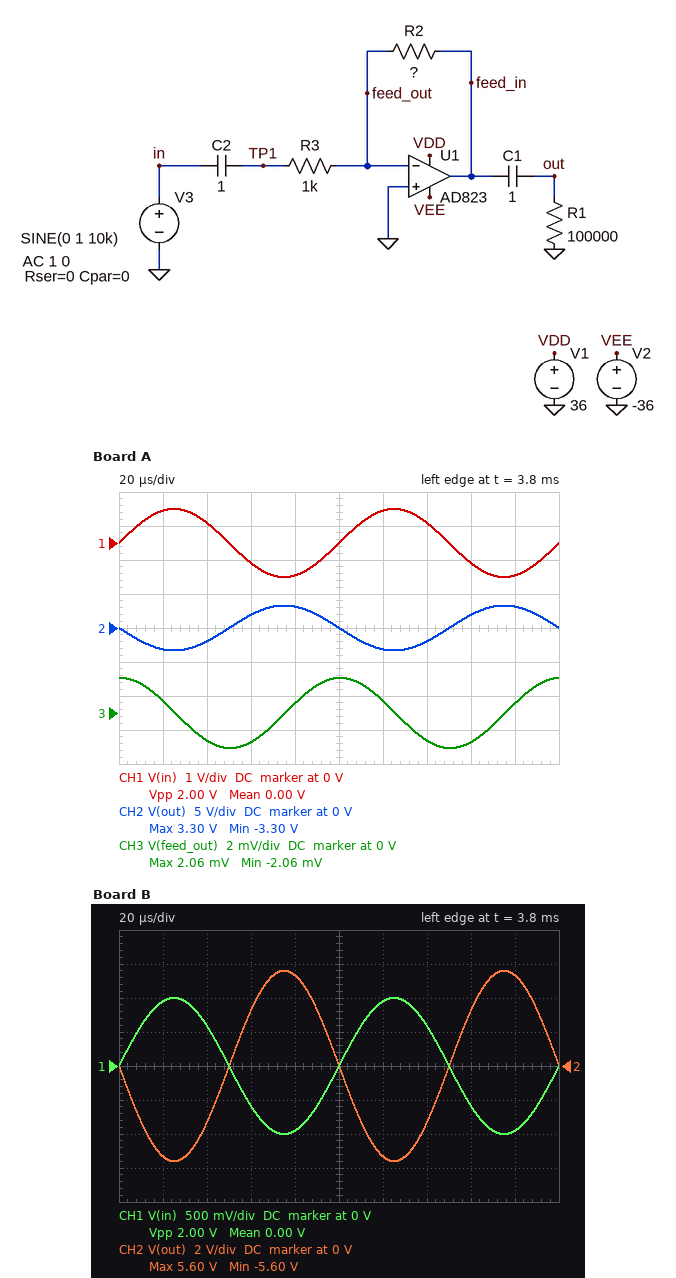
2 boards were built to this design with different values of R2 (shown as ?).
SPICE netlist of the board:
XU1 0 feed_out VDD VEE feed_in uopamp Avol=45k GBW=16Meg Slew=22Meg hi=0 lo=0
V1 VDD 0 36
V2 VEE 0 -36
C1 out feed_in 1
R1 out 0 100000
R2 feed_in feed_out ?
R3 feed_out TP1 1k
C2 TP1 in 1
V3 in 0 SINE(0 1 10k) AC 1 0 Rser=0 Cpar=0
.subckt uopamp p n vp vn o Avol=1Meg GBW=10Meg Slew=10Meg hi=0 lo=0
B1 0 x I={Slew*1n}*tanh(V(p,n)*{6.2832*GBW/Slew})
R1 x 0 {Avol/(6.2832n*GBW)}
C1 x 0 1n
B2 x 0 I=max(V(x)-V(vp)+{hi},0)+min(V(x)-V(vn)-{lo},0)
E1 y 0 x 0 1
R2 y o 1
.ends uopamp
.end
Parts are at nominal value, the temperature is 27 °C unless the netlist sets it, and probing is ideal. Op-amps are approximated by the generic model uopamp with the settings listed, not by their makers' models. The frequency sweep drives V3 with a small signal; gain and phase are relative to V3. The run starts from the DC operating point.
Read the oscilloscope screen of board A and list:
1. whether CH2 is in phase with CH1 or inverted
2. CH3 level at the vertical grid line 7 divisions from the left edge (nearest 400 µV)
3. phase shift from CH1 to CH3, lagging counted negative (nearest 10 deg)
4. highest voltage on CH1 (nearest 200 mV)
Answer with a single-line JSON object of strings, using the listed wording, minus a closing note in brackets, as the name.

{"whether CH2 is in phase with CH1 or inverted": "inverted", "CH3 level at the vertical grid line 7 divisions from the left edge": "-1.6 mV", "phase shift from CH1 to CH3, lagging counted negative": "90 deg", "highest voltage on CH1": "1.0 V"}
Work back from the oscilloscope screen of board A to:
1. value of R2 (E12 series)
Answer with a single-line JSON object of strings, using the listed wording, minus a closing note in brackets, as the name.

{"value of R2": "3.3 kΩ"}
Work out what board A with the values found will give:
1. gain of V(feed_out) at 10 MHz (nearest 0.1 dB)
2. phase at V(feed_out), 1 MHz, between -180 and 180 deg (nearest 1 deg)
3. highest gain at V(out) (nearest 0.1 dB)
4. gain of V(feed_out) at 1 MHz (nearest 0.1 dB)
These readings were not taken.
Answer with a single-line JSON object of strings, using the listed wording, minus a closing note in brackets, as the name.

{"gain of V(feed_out) at 10 MHz": "-2.9 dB", "phase at V(feed_out), 1 MHz, between -180 and 180 deg": "75 deg", "highest gain at V(out)": "10.4 dB", "gain of V(feed_out) at 1 MHz": "-14.0 dB"}
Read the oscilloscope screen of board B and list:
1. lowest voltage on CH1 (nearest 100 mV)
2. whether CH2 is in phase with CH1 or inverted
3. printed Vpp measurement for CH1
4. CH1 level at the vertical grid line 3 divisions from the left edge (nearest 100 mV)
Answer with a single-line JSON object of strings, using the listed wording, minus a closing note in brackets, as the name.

{"lowest voltage on CH1": "-1.0 V", "whether CH2 is in phase with CH1 or inverted": "inverted", "printed Vpp measurement for CH1": "2.00 V", "CH1 level at the vertical grid line 3 divisions from the left edge": "-600 mV"}
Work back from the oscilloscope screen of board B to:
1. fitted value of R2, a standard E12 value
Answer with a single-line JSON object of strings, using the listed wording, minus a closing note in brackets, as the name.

{"fitted value of R2, a standard E12 value": "5.6 kΩ"}
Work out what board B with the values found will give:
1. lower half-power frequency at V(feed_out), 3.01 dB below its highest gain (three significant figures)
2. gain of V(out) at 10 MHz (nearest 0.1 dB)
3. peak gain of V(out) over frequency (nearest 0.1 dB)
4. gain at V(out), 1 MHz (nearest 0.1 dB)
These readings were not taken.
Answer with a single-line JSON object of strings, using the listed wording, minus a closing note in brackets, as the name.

{"lower half-power frequency at V(feed_out), 3.01 dB below its highest gain": "2.42 MHz", "gain of V(out) at 10 MHz": "2.4 dB", "peak gain of V(out) over frequency": "15.0 dB", "gain at V(out), 1 MHz": "14.3 dB"}
